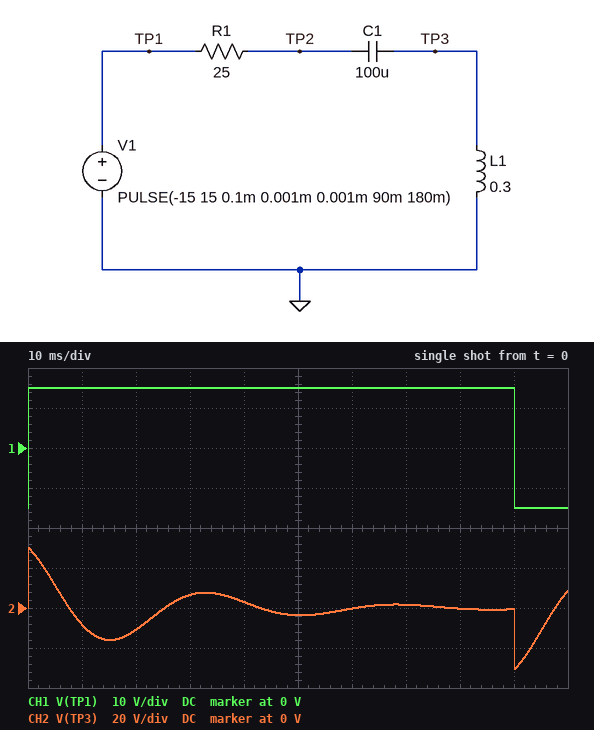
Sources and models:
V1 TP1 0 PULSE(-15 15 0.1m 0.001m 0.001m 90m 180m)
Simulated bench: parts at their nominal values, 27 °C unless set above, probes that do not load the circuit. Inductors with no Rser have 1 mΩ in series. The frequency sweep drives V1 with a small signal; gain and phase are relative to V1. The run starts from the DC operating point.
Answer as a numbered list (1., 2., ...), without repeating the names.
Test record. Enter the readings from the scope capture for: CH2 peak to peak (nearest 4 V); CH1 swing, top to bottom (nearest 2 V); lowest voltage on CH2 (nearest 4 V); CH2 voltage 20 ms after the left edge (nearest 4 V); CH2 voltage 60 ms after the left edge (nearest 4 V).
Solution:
1. 60 V
2. 30 V
3. -32 V
4. -12 V
5. 0 V
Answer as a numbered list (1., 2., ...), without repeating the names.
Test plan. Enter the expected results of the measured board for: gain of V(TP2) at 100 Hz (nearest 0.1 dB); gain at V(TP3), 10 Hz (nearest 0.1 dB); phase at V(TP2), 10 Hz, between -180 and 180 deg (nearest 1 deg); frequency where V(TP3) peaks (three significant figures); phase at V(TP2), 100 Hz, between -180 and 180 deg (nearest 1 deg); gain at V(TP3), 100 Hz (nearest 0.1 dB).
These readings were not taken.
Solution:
1. -0.1 dB
2. -17.6 dB
3. -10 deg
4. 30.7 Hz
5. 8 deg
6. 0.7 dB
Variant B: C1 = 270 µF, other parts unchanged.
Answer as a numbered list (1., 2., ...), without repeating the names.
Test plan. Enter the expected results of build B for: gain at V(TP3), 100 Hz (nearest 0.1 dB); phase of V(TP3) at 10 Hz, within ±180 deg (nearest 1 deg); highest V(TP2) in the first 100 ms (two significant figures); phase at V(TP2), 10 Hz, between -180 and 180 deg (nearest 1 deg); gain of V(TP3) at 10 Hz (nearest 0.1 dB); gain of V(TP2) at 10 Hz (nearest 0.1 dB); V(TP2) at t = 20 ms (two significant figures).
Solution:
1. 0.2 dB
2. 148 deg
3. 19 V
4. -32 deg
5. -8.0 dB
6. -1.4 dB
7. 5.6 V
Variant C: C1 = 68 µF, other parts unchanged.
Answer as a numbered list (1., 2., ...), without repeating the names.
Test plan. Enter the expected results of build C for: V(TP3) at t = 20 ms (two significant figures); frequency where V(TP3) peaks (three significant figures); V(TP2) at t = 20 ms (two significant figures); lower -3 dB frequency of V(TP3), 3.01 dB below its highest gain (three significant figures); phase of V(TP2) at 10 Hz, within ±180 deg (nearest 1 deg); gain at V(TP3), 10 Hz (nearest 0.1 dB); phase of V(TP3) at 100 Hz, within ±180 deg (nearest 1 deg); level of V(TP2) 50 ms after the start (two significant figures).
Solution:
1. -2.6 V
2. 36.6 Hz
3. 20 V
4. 30.9 Hz
5. -7 deg
6. -21.2 dB
7. 9 deg
8. 16 V
